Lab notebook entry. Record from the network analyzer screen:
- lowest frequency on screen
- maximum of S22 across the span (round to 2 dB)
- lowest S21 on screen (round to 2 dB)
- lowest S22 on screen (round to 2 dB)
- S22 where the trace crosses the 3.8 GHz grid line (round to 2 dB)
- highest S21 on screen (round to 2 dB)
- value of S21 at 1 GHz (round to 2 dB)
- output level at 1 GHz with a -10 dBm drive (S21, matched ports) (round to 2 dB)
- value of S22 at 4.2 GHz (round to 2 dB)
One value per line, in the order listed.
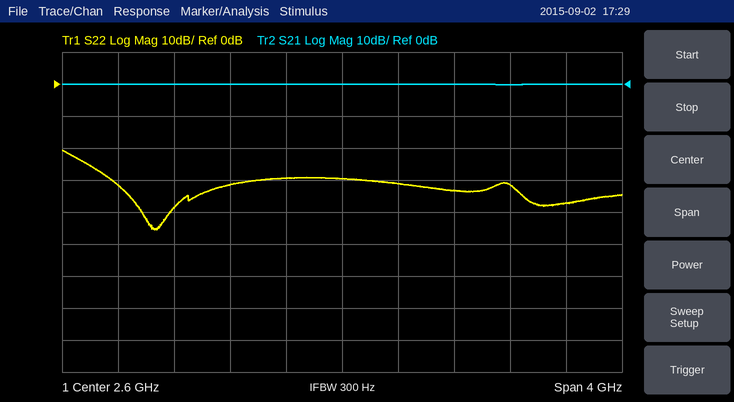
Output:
600 MHz
-20 dB
0 dB
-46 dB
-32 dB
0 dB
0 dB
-10 dBm
-38 dB
